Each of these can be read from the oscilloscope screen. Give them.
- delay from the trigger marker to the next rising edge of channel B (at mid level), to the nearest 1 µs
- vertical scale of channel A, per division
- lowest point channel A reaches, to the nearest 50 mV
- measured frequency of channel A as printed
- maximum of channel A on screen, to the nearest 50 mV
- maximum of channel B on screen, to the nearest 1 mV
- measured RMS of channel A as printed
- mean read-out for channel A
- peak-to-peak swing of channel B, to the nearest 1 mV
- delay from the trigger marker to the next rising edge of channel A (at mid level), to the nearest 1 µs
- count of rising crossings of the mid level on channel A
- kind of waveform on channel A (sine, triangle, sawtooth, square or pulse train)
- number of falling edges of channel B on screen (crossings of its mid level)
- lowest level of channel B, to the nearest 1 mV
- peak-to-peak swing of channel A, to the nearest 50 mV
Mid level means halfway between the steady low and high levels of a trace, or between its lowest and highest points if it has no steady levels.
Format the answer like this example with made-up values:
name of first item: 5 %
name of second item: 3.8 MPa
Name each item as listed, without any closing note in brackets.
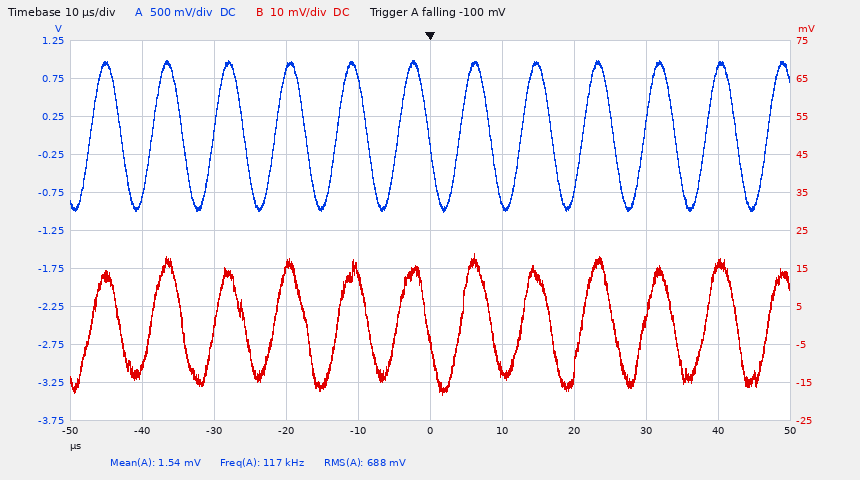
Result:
delay from the trigger marker to the next rising edge of channel B (at mid level), to the nearest 1 µs: 4 µs
vertical scale of channel A, per division: 500 mV
lowest point channel A reaches, to the nearest 50 mV: -1.00 V
measured frequency of channel A as printed: 117 kHz
maximum of channel A on screen, to the nearest 50 mV: 1.00 V
maximum of channel B on screen, to the nearest 1 mV: 19 mV
measured RMS of channel A as printed: 688 mV
mean read-out for channel A: 1.54 mV
peak-to-peak swing of channel B, to the nearest 1 mV: 37 mV
delay from the trigger marker to the next rising edge of channel A (at mid level), to the nearest 1 µs: 4 µs
count of rising crossings of the mid level on channel A: 12
kind of waveform on channel A: sine
number of falling edges of channel B on screen: 11
lowest level of channel B, to the nearest 1 mV: -18 mV
peak-to-peak swing of channel A, to the nearest 50 mV: 2.00 V
